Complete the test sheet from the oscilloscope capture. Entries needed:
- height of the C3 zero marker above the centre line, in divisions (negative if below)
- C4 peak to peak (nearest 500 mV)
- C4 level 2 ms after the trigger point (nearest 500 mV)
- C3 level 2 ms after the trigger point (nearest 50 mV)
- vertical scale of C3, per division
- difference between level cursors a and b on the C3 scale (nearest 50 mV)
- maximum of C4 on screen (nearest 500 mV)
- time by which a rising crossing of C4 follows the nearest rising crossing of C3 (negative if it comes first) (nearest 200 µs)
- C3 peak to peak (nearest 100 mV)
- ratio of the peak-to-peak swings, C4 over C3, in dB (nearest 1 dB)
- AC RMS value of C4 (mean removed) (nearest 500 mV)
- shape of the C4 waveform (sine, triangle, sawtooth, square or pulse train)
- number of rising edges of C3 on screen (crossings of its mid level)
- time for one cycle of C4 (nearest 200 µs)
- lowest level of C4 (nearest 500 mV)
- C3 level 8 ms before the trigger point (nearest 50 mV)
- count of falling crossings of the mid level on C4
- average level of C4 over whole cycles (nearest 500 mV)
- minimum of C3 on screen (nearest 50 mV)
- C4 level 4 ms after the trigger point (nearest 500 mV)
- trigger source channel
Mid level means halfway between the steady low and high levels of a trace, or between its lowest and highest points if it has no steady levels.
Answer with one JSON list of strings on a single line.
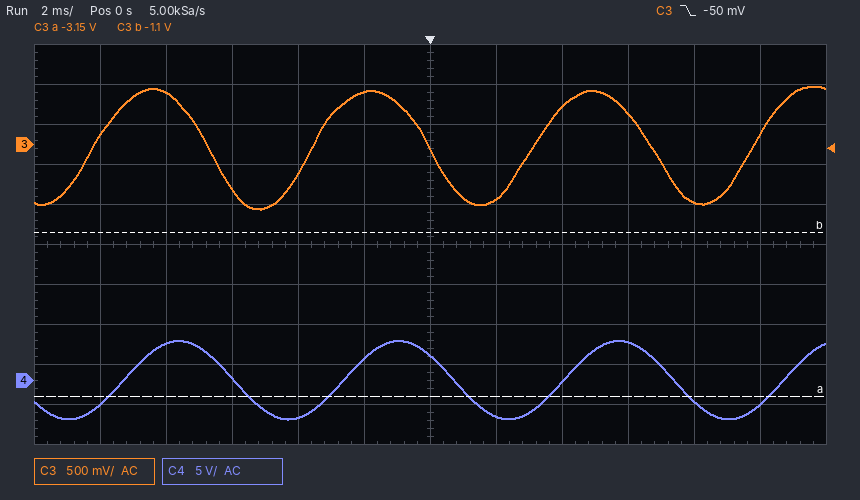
["+2.5 div", "10.0 V", "-4.5 V", "-700 mV", "500 mV", "2.05 V", "5.0 V", "+1.0 ms", "1.50 V", "16 dB", "3.5 V", "sine", "4", "6.6 ms", "-5.0 V", "650 mV", "3", "0.0 V", "-800 mV", "0.0 V", "C3"]
